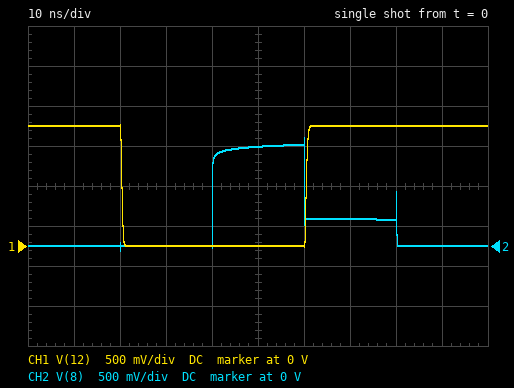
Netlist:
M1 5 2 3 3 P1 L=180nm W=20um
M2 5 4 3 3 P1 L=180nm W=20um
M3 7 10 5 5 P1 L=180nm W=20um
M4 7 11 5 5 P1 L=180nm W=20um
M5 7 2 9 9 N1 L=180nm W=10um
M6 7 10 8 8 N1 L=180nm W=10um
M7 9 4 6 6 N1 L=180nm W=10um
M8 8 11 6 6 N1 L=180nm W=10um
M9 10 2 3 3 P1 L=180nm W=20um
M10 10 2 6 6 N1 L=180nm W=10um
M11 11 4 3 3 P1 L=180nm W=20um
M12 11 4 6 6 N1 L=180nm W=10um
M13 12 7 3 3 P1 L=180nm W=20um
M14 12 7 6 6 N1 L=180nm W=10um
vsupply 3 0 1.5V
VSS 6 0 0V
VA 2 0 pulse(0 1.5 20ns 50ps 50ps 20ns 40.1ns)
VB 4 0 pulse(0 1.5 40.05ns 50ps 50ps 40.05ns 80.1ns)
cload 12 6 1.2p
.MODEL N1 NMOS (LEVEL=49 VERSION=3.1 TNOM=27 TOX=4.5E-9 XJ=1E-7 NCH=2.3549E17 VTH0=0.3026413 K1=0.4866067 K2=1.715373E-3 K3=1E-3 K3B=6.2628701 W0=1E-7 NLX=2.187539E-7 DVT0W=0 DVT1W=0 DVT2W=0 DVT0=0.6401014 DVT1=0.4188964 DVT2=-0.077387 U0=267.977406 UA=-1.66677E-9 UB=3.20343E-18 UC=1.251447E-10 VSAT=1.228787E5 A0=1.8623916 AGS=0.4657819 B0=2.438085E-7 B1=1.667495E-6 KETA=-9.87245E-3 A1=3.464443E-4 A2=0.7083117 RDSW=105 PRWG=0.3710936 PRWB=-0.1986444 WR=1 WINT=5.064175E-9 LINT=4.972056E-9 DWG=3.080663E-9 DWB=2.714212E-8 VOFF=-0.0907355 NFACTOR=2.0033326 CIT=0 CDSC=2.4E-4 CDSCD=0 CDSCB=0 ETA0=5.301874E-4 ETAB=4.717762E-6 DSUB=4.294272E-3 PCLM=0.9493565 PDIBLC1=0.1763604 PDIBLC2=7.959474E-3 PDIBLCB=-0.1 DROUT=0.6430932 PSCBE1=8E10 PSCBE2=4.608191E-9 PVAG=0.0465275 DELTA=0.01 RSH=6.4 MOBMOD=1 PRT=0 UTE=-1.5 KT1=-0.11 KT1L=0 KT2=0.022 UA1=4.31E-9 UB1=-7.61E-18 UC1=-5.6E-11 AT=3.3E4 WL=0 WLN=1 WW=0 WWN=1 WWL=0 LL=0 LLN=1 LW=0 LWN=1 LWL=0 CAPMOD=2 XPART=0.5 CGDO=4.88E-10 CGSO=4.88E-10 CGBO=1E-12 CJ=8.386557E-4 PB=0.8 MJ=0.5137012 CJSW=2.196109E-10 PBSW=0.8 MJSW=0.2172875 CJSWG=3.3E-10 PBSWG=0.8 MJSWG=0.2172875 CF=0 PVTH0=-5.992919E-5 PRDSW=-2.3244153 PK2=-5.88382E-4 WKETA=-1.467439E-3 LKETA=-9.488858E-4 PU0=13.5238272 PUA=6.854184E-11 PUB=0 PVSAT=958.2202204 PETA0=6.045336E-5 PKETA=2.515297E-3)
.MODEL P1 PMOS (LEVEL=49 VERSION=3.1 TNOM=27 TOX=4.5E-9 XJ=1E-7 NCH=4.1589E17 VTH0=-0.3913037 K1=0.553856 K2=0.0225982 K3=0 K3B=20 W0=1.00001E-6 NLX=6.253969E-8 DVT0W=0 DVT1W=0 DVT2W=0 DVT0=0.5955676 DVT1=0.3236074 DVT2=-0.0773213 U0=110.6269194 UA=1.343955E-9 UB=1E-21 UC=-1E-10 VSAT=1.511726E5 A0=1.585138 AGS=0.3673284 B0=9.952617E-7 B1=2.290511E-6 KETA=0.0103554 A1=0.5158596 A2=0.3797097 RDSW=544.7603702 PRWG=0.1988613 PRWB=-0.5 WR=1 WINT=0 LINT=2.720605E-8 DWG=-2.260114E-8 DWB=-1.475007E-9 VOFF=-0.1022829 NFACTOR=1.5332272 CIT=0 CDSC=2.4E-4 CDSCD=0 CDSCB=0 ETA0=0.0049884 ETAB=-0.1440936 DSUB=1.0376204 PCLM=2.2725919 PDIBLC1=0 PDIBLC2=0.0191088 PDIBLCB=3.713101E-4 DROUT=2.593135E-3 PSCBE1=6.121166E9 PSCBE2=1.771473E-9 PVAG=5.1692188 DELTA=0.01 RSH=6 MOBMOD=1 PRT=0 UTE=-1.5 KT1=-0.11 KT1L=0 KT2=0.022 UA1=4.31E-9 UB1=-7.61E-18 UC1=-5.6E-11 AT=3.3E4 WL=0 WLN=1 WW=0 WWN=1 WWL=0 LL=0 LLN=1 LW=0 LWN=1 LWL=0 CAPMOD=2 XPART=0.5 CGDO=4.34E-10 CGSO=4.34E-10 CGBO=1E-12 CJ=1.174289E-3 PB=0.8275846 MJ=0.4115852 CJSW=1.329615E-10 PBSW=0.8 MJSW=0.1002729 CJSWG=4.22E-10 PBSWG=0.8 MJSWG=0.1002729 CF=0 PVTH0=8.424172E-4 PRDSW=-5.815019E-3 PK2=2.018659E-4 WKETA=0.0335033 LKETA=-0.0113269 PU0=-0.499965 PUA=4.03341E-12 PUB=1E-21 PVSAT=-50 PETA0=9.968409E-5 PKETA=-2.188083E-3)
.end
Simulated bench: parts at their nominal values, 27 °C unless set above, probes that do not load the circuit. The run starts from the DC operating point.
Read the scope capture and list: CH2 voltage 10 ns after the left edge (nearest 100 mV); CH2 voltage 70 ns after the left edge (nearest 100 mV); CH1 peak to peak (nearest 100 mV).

0 V
300 mV
1.5 V
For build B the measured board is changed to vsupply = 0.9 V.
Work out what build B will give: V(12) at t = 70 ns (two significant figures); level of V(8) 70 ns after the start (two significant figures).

900 mV
100 mV
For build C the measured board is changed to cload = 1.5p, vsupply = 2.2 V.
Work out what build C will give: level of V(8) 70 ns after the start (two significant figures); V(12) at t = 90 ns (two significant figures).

520 mV
2.2 V
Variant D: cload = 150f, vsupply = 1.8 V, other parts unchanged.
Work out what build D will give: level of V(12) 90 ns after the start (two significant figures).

1.8 V
